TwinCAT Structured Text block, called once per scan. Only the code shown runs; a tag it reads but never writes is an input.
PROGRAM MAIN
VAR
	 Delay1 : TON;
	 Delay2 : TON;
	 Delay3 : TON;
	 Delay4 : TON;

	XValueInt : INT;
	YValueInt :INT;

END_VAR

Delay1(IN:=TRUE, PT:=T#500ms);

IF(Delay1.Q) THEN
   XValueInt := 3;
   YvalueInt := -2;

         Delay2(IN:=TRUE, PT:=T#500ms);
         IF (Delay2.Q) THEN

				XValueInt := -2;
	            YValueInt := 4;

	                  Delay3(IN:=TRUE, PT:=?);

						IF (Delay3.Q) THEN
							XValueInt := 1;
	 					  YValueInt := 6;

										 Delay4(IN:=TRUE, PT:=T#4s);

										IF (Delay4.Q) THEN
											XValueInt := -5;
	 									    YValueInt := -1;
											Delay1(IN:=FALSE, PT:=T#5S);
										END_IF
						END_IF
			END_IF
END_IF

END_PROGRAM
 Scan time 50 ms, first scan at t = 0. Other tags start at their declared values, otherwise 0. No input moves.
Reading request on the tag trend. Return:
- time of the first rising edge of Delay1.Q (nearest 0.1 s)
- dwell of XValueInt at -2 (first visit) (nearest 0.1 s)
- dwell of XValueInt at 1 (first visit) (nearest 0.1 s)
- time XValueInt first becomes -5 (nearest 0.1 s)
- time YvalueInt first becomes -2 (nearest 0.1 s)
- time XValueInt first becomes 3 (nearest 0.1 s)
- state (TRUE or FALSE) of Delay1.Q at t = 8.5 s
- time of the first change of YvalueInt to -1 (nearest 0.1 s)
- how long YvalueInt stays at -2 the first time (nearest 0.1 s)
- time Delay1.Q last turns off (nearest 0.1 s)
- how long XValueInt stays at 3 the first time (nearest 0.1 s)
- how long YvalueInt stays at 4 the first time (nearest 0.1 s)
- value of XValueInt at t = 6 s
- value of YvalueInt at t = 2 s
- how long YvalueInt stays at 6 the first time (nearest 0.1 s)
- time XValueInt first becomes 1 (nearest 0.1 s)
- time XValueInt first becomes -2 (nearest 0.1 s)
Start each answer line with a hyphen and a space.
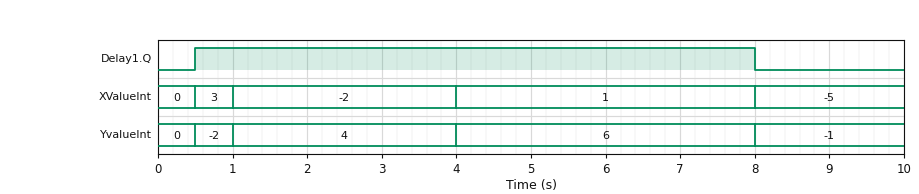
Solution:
- 0.5 s
- 3.0 s
- 4.0 s
- 8.0 s
- 0.5 s
- 0.5 s
- FALSE
- 8.0 s
- 0.5 s
- 8.0 s
- 0.5 s
- 3.0 s
- 1
- 4
- 4.0 s
- 4.0 s
- 1.0 s
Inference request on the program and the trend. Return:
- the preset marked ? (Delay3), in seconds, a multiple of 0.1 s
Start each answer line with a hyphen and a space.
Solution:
- 3.0 s
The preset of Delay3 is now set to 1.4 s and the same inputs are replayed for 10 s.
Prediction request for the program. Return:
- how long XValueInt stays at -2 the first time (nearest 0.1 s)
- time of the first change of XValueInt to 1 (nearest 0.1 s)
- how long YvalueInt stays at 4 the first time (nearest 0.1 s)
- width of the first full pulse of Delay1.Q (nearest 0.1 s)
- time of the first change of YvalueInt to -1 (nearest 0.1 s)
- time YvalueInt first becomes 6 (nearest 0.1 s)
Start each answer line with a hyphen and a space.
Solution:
- 1.4 s
- 2.4 s
- 1.4 s
- 5.9 s
- 6.4 s
- 2.4 s
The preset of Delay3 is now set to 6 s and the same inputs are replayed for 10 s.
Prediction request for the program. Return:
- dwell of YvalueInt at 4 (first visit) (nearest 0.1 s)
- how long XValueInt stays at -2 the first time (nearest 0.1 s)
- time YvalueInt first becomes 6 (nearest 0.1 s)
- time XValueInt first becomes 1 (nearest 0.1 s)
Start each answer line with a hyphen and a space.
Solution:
- 6.0 s
- 6.0 s
- 7.0 s
- 7.0 s
